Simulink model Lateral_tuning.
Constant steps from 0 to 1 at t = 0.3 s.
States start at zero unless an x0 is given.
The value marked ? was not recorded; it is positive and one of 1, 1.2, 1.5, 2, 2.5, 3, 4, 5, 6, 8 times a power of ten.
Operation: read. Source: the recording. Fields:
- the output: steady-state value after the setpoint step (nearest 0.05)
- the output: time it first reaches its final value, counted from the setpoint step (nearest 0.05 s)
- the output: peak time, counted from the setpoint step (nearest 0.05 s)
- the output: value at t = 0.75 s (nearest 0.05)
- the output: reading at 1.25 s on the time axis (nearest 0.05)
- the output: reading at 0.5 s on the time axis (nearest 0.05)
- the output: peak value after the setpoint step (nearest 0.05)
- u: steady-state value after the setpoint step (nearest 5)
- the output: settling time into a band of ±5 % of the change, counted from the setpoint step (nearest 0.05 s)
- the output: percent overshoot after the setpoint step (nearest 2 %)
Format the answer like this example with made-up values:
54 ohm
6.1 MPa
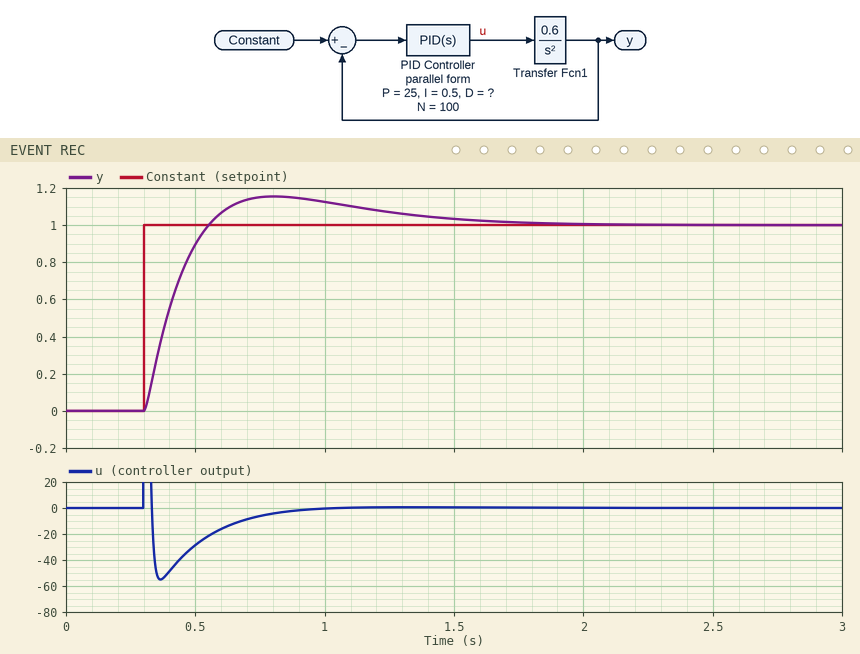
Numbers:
1.00
0.25 s
0.50 s
1.15
1.05
0.90
1.15
0
1.05 s
16 %
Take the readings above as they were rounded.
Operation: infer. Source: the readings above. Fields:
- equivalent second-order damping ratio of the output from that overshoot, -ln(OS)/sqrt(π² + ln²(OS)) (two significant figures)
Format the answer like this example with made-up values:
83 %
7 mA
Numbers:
0.50
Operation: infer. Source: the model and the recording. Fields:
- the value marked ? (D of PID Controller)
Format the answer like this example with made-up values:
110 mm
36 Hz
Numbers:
12
